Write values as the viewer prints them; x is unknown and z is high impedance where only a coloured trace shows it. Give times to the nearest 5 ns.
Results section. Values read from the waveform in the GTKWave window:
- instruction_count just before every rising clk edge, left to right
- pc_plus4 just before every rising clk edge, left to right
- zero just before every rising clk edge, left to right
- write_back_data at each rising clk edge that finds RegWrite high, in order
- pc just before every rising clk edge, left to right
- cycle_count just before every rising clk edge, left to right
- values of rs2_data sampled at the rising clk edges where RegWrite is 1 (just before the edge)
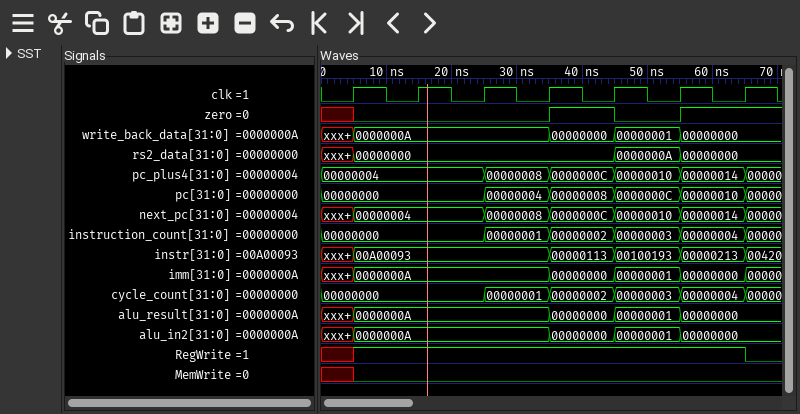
00000000, 00000000, 00000000, 00000001, 00000002, 00000003, 00000004
00000004, 00000004, 00000004, 00000008, 0000000C, 00000010, 00000014
x 0 0 0 1 0 1
0000000A, 0000000A, 0000000A, 00000000, 00000001, 00000000
00000000, 00000000, 00000000, 00000004, 00000008, 0000000C, 00000010
00000000, 00000000, 00000000, 00000001, 00000002, 00000003, 00000004
00000000, 00000000, 00000000, 00000000, 0000000A, 00000000
